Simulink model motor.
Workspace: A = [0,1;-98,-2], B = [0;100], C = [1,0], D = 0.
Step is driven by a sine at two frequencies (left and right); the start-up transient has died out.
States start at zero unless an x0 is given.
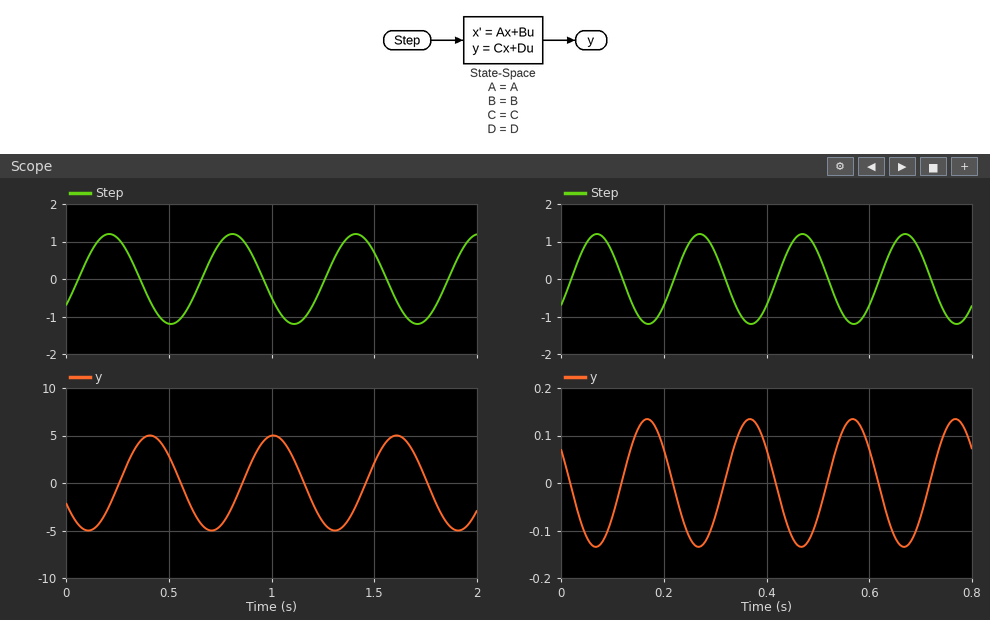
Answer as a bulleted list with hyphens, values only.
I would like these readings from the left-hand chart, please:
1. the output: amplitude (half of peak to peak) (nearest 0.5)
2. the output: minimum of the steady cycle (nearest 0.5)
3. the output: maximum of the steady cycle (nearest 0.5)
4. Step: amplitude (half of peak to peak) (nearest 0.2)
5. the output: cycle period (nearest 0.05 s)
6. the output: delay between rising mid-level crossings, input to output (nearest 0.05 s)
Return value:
- 5.0
- -5.0
- 5.0
- 1.2
- 0.60 s
- 0.20 s
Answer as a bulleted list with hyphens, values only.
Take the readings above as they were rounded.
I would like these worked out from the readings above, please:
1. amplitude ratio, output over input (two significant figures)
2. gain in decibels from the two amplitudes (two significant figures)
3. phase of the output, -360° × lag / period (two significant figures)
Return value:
- 4.2
- 12 dB
- -120°
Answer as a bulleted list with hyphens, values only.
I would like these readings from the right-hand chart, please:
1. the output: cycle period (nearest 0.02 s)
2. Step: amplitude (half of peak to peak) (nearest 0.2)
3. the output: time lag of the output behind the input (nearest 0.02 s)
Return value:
- 0.20 s
- 1.2
- 0.10 s
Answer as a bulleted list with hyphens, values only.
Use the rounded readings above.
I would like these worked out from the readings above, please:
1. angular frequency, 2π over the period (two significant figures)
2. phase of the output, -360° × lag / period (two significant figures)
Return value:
- 31 rad/s
- -180°
